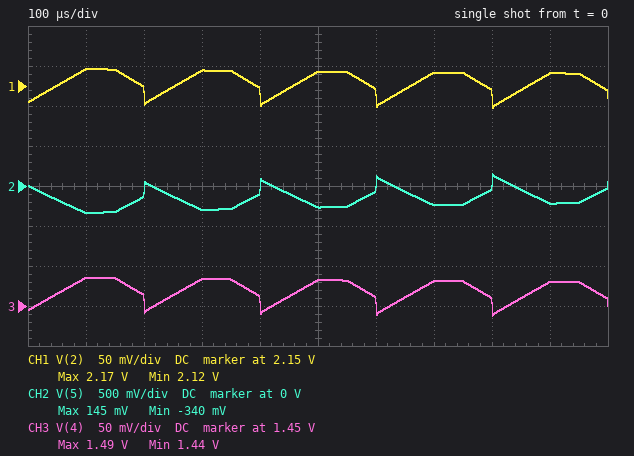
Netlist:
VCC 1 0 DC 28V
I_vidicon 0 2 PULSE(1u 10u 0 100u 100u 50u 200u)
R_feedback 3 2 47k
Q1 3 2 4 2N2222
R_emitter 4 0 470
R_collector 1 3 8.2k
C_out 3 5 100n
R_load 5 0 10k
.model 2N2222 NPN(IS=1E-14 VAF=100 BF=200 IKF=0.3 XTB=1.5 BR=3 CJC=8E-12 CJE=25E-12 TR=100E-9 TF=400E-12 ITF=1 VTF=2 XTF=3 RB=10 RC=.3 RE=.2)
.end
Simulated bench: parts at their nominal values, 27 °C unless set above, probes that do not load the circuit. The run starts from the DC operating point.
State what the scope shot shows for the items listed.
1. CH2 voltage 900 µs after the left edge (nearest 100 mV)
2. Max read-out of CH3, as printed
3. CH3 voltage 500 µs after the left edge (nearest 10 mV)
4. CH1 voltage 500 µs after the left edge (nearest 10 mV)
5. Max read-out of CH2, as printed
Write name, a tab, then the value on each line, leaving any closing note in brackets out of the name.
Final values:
CH2 voltage 900 µs after the left edge	-200 mV
Max read-out of CH3, as printed	1.49 V
CH3 voltage 500 µs after the left edge	1.48 V
CH1 voltage 500 µs after the left edge	2.17 V
Max read-out of CH2, as printed	145 mV
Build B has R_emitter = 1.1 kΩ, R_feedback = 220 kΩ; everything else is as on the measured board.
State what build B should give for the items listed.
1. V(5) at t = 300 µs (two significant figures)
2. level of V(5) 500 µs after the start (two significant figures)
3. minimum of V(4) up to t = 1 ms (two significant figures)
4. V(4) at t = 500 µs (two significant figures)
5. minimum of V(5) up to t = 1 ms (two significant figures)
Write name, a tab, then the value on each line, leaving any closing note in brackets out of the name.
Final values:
V(5) at t = 300 µs	-1.1 V
level of V(5) 500 µs after the start	-980 mV
minimum of V(4) up to t = 1 ms	2.9 V
V(4) at t = 500 µs	3.2 V
minimum of V(5) up to t = 1 ms	-1.2 V
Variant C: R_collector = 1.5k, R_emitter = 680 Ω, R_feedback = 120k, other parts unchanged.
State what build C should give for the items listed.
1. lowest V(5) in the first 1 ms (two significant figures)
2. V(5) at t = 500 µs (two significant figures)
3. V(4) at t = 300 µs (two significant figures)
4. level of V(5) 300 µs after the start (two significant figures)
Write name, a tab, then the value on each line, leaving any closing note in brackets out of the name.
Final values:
lowest V(5) in the first 1 ms	-490 mV
V(5) at t = 500 µs	-390 mV
V(4) at t = 300 µs	7.0 V
level of V(5) 300 µs after the start	-430 mV
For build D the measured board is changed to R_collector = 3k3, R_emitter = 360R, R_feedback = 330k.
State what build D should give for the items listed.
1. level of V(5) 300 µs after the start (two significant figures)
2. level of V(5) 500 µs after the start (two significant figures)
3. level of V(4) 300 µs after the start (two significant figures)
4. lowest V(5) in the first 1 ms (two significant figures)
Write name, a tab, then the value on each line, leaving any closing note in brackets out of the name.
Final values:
level of V(5) 300 µs after the start	-1.3 V
level of V(5) 500 µs after the start	-1.2 V
level of V(4) 300 µs after the start	2.1 V
lowest V(5) in the first 1 ms	-1.5 V
